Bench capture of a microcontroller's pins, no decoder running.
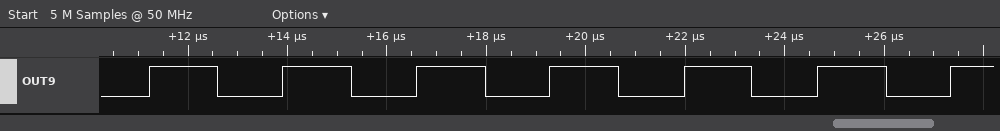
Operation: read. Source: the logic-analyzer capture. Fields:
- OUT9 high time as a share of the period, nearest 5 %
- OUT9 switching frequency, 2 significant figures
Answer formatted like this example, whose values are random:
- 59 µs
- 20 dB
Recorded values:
- 50 %
- 370 kHz
